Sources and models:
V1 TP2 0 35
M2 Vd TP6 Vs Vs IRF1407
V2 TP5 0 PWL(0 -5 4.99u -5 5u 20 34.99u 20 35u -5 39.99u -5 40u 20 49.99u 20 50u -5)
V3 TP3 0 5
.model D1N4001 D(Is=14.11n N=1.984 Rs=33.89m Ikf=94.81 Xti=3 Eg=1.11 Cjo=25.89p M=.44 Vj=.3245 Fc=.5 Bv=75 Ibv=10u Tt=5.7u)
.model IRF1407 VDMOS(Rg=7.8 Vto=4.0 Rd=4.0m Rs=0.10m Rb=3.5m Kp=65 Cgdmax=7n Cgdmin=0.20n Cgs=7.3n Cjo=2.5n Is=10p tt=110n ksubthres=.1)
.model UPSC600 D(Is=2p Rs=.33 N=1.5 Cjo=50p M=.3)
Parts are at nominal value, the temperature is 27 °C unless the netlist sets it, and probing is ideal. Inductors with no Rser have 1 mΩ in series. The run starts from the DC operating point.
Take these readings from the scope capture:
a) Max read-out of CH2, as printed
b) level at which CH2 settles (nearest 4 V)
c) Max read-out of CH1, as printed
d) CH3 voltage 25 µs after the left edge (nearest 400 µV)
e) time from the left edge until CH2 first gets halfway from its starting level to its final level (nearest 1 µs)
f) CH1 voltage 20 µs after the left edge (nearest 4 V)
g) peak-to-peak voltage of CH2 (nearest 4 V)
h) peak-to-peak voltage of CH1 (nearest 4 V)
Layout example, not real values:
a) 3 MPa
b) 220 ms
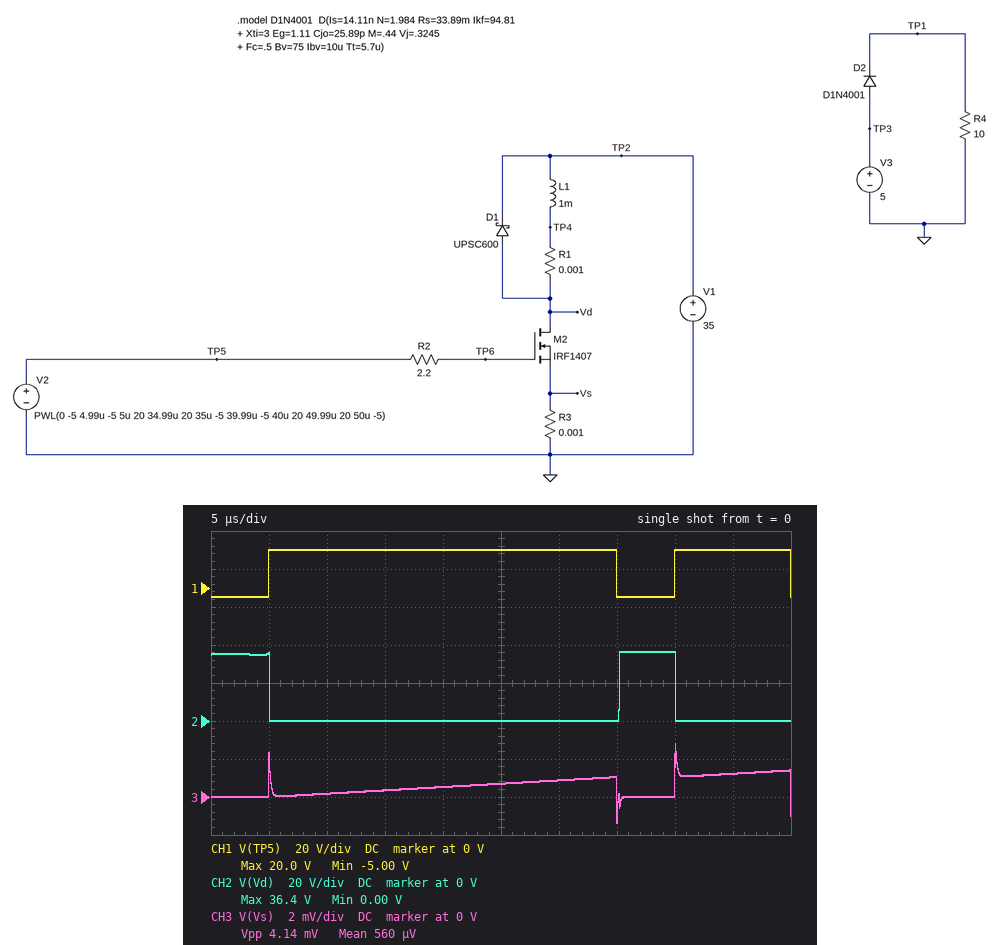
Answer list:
a) 36.4 V
b) 0 V
c) 20.0 V
d) 800 µV
e) 5 µs
f) 20 V
g) 36 V
h) 24 V
